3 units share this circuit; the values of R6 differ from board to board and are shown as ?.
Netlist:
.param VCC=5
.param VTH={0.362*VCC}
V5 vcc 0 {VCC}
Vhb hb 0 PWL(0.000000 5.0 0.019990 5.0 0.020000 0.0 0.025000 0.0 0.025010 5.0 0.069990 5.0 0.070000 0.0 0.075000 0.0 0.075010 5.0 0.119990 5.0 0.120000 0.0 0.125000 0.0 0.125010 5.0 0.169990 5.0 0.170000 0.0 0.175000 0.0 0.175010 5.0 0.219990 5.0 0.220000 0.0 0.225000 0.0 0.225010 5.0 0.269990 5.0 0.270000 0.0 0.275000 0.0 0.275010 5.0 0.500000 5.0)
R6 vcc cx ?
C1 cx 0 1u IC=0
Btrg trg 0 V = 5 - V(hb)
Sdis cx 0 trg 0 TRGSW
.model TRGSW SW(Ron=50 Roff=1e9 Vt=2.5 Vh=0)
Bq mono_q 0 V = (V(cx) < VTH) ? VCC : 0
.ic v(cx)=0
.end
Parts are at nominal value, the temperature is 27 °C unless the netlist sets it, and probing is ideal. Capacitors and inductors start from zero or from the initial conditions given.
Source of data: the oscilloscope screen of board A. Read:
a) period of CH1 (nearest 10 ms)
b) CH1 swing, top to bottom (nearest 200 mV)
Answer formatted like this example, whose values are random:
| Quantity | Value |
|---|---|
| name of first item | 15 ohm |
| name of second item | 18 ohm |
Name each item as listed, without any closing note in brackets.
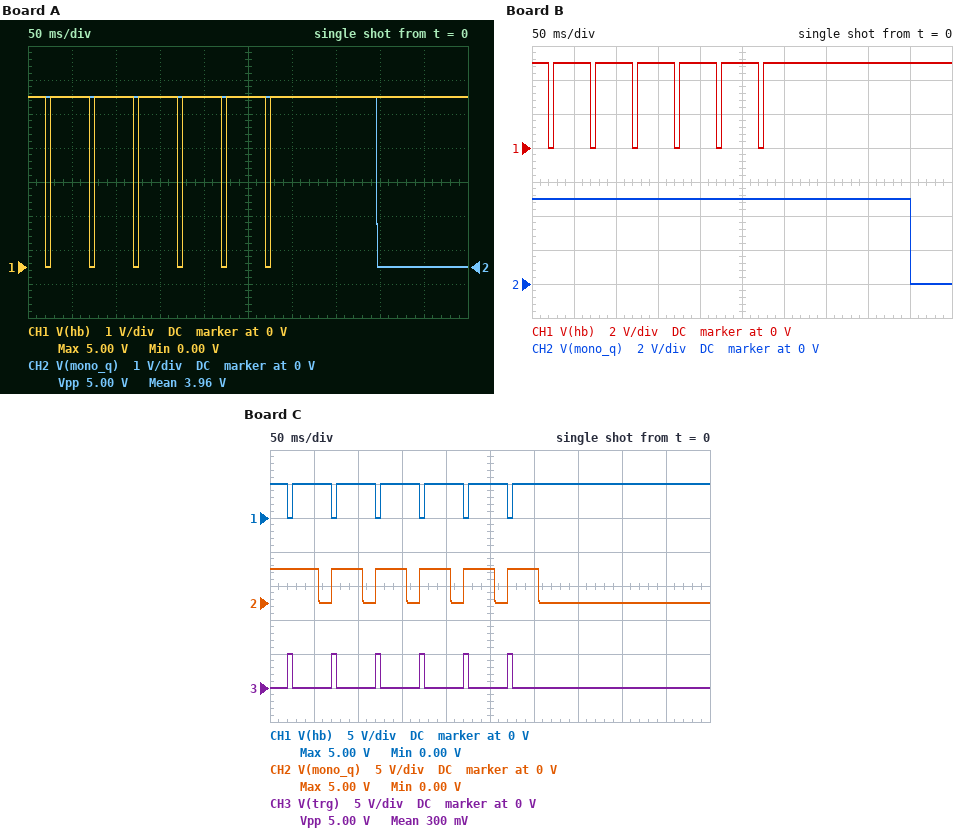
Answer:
| Quantity | Value |
|---|---|
| period of CH1 | 50 ms |
| CH1 swing, top to bottom | 5.0 V |
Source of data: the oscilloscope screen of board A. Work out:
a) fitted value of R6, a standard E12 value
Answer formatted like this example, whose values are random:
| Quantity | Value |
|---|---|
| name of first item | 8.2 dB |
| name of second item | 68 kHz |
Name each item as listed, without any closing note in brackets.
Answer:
| Quantity | Value |
|---|---|
| fitted value of R6, a standard E12 value | 270 kΩ |
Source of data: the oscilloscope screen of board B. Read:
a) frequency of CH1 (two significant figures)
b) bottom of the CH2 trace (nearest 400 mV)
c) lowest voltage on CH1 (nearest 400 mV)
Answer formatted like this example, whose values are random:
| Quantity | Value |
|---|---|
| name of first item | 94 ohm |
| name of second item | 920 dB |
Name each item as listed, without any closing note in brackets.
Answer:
| Quantity | Value |
|---|---|
| frequency of CH1 | 20 Hz |
| bottom of the CH2 trace | 0 V |
| lowest voltage on CH1 | 0 V |
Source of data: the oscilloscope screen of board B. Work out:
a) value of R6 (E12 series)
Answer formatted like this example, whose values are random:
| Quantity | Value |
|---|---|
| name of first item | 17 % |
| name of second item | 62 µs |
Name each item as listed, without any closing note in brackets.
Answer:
| Quantity | Value |
|---|---|
| value of R6 | 390 kΩ |
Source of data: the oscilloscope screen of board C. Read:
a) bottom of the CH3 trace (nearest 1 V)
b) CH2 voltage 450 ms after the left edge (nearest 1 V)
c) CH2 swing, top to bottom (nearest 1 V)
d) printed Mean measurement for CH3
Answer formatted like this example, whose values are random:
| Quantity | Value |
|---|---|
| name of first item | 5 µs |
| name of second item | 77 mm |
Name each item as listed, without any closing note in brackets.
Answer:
| Quantity | Value |
|---|---|
| bottom of the CH3 trace | 0 V |
| CH2 voltage 450 ms after the left edge | 0 V |
| CH2 swing, top to bottom | 5 V |
| printed Mean measurement for CH3 | 300 mV |
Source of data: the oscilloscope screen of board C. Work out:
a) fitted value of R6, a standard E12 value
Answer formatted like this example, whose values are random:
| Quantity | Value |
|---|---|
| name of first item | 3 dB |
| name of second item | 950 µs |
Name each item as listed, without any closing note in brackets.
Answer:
| Quantity | Value |
|---|---|
| fitted value of R6, a standard E12 value | 68 kΩ |
